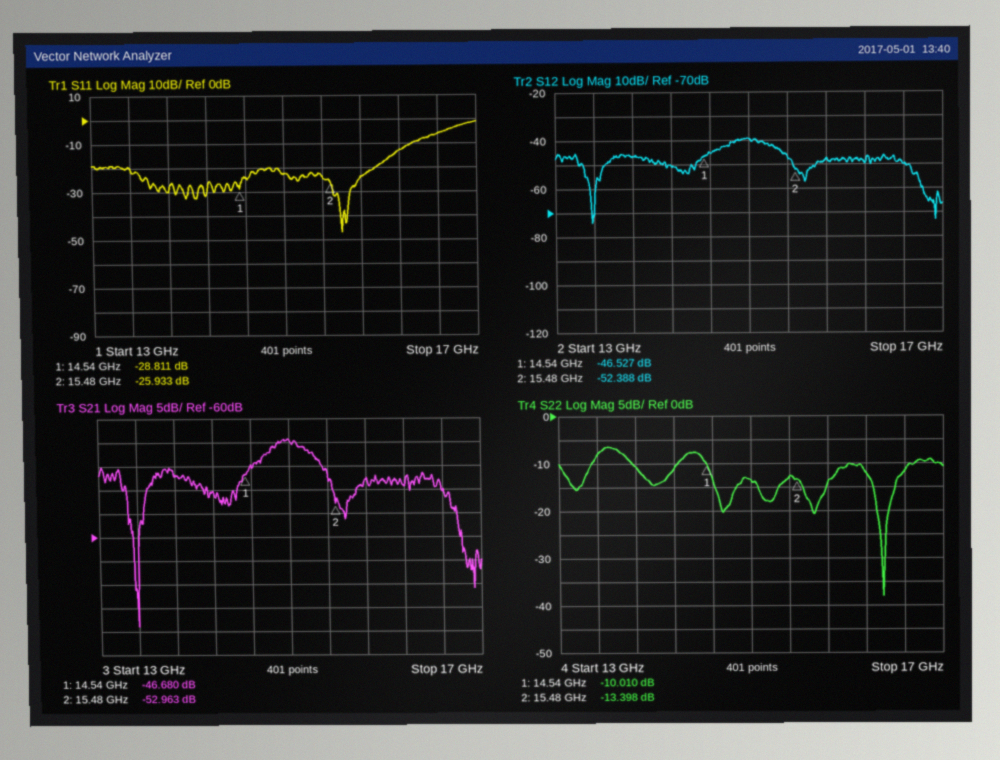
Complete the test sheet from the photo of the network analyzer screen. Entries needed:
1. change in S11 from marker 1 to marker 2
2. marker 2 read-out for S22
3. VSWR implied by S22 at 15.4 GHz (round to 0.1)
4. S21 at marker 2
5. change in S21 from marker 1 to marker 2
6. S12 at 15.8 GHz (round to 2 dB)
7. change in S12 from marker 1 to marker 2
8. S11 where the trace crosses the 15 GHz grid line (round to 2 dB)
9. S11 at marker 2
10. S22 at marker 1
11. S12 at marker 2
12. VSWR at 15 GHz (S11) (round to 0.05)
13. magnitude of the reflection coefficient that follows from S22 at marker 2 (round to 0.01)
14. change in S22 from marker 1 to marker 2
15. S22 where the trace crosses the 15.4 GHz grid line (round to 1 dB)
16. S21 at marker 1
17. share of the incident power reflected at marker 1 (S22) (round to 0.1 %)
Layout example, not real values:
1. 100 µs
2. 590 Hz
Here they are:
1. 2.878 dB
2. -13.398 dB
3. 1.6
4. -52.963 dB
5. -6.283 dB
6. -48 dB
7. -5.861 dB
8. -22 dB
9. -25.933 dB
10. -10.010 dB
11. -52.388 dB
12. 1.15
13. 0.21
14. -3.388 dB
15. -13 dB
16. -46.680 dB
17. 10.0 %
